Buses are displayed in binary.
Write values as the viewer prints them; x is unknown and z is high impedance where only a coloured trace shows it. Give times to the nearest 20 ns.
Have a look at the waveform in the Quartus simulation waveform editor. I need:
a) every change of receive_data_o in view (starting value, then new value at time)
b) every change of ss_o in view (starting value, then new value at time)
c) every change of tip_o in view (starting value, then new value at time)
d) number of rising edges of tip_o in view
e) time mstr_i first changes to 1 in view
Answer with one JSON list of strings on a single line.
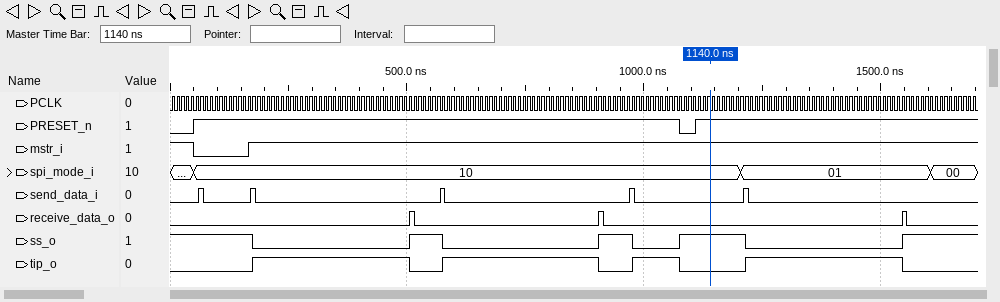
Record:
["0, 1 at 500 ns, 0 at 520 ns, 1 at 900 ns, 0 at 920 ns, 1 at 1540 ns, 0 at 1560 ns", "1, 0 at 180 ns, 1 at 500 ns, 0 at 580 ns, 1 at 900 ns, 0 at 980 ns, 1 at 1080 ns, 0 at 1220 ns, 1 at 1540 ns", "0, 1 at 180 ns, 0 at 500 ns, 1 at 580 ns, 0 at 900 ns, 1 at 980 ns, 0 at 1080 ns, 1 at 1220 ns, 0 at 1540 ns", "4", "160 ns"]
